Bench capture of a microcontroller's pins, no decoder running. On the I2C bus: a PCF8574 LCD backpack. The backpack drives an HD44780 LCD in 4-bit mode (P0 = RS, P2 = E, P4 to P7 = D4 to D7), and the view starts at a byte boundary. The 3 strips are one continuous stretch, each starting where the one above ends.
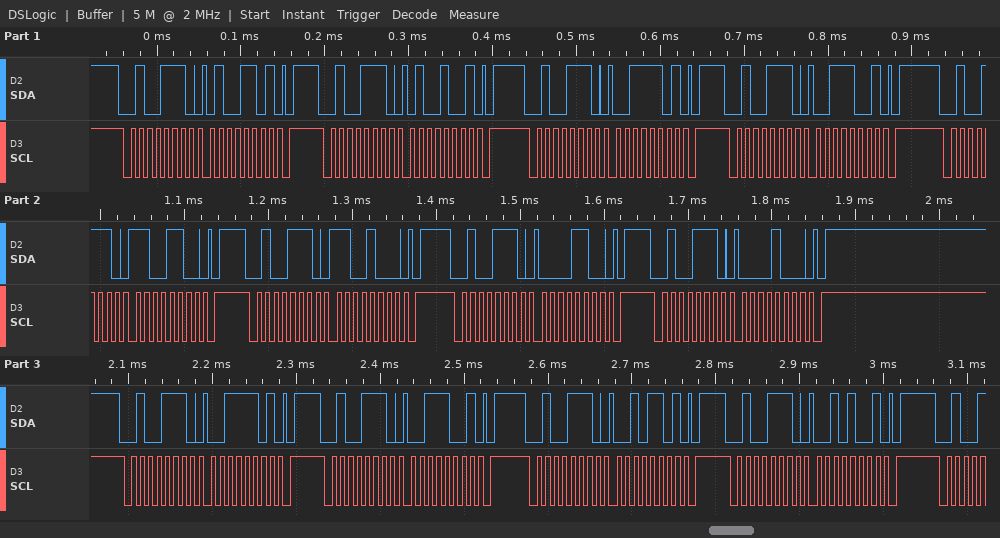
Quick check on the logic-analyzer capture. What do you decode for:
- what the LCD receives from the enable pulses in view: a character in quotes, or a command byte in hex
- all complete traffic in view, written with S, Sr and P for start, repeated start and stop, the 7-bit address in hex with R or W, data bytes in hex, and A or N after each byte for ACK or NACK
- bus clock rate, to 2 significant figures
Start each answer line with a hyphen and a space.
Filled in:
- 'C' 0xC0 '2'
- S 27W A 4D A P S 27W A 49 A P S 27W A 3D A P S 27W A 39 A P S 27W A CC A P S 27W A C8 A P S 27W A 0C A P S 27W A 08 A P S 27W A 3D A P S 27W A 39 A P S 27W A 2D A P S 27W A 29 A P
- 100 kHz
